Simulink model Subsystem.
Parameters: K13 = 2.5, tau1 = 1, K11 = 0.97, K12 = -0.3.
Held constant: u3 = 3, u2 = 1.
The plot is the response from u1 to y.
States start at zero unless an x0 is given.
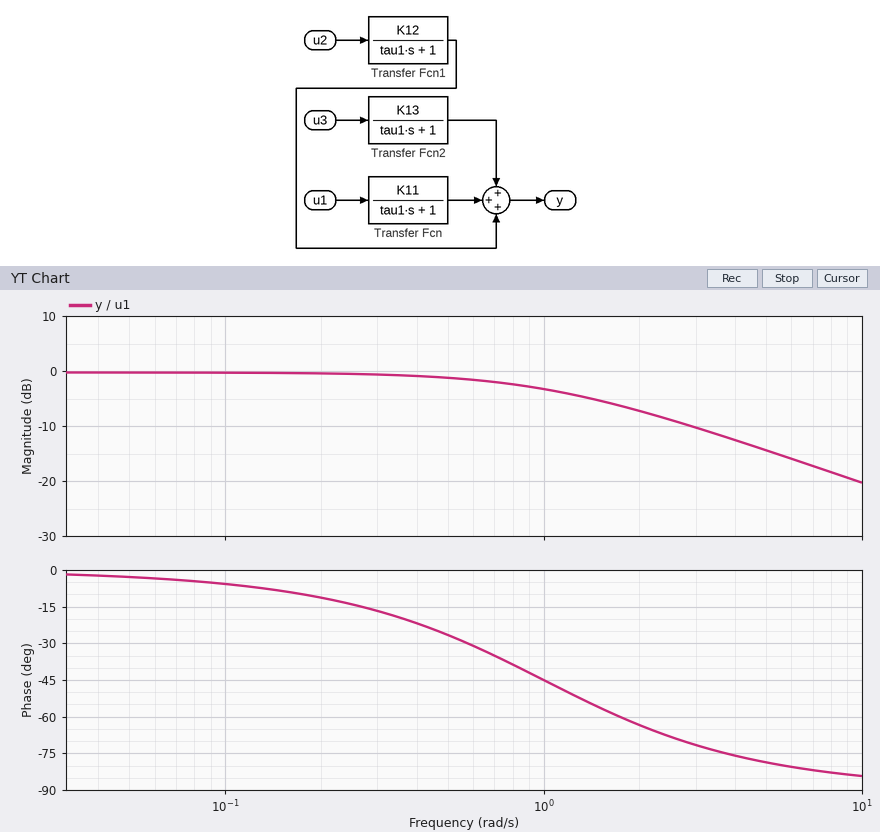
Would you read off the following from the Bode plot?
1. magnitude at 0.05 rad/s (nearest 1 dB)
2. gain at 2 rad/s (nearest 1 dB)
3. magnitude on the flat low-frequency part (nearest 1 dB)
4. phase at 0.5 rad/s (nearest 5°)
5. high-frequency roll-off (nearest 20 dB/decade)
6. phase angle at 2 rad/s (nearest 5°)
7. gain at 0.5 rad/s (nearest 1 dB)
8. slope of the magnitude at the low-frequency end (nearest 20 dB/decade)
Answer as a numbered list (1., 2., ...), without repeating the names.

1. 0 dB
2. -7 dB
3. 0 dB
4. -25°
5. -20 dB/decade
6. -65°
7. -1 dB
8. 0 dB/decade
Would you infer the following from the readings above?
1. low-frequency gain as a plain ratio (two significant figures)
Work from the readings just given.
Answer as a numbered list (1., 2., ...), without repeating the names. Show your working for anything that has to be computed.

1. 10^(0 / 20) = 1.0
